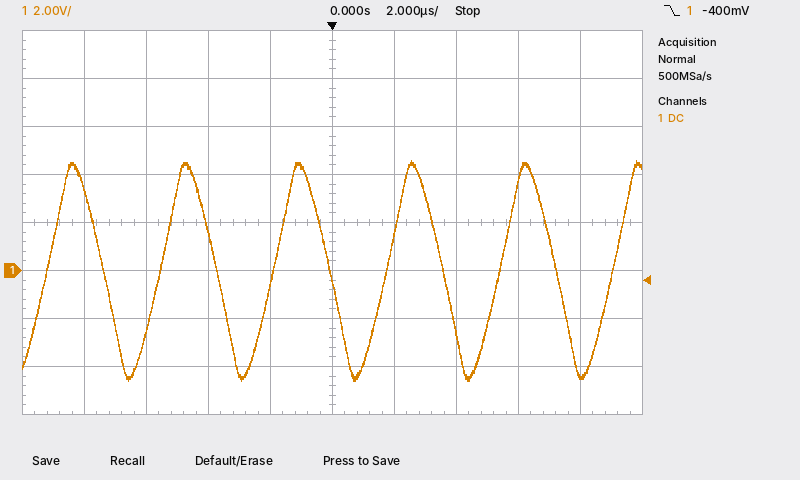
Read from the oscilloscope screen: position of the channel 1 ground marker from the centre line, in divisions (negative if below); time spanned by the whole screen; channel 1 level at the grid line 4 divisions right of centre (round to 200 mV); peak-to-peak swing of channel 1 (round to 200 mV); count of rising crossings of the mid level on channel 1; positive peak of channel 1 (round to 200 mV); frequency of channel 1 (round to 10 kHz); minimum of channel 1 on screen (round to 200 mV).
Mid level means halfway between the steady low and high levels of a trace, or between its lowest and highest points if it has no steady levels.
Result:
-1.0 div
20 µs
-4.4 V
9.2 V
6
4.6 V
270 kHz
-4.6 V
